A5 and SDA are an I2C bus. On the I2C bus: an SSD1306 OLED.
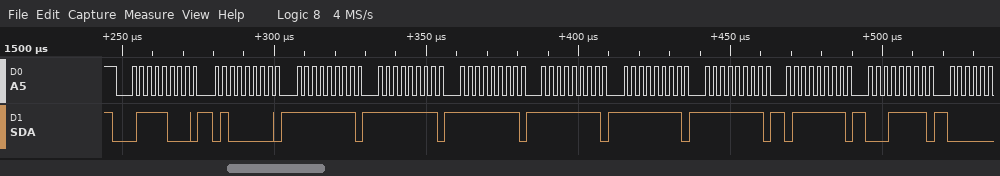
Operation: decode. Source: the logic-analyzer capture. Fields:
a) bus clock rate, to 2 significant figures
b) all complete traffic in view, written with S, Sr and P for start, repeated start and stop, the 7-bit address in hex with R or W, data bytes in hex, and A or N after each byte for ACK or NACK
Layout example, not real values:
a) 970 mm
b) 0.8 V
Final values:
a) 400 kHz
b) S 3CW A 40 A FF A FF A FF A FF A FF A FF A 7F A 1F A
